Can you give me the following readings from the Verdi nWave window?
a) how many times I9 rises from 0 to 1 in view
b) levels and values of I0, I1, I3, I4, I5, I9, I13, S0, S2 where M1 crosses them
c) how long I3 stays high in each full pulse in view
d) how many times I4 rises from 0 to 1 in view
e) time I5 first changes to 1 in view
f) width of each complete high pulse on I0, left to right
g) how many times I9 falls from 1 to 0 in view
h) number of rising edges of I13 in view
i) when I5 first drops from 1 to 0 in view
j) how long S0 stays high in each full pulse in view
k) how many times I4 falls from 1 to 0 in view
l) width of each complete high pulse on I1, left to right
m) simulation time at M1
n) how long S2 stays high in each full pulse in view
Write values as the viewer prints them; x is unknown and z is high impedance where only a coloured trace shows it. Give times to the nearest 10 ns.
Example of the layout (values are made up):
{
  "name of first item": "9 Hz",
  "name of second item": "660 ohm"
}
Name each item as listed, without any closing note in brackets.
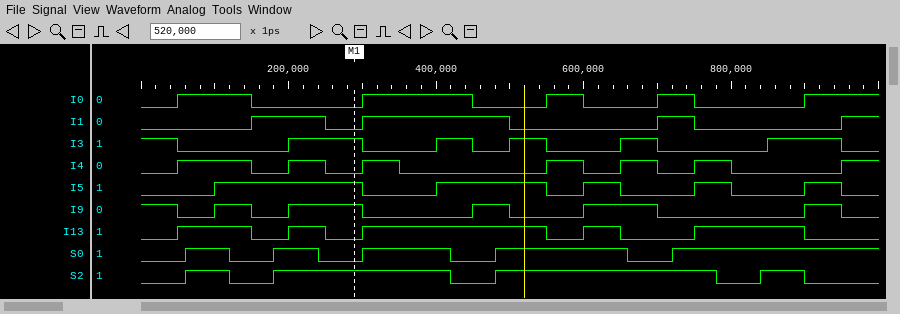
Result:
{
  "how many times I9 rises from 0 to 1 in view": "5",
  "levels and values of I0, I1, I3, I4, I5, I9, I13, S0, S2 where M1 crosses them": "I0=0, I1=0, I3=1, I4=0, I5=1, I9=1, I13=0, S0=0, S2=1",
  "how long I3 stays high in each full pulse in view": "100 ns, 50 ns, 50 ns, 50 ns, 100 ns",
  "how many times I4 rises from 0 to 1 in view": "7",
  "time I5 first changes to 1 in view": "100 ns",
  "width of each complete high pulse on I0, left to right": "100 ns, 150 ns, 50 ns, 50 ns",
  "how many times I9 falls from 1 to 0 in view": "6",
  "number of rising edges of I13 in view": "5",
  "when I5 first drops from 1 to 0 in view": "300 ns",
  "how long S0 stays high in each full pulse in view": "60 ns, 60 ns, 120 ns, 180 ns",
  "how many times I4 falls from 1 to 0 in view": "6",
  "width of each complete high pulse on I1, left to right": "100 ns, 200 ns, 50 ns",
  "simulation time at M1": "290 ns",
  "how long S2 stays high in each full pulse in view": "60 ns, 240 ns, 300 ns, 60 ns"
}
